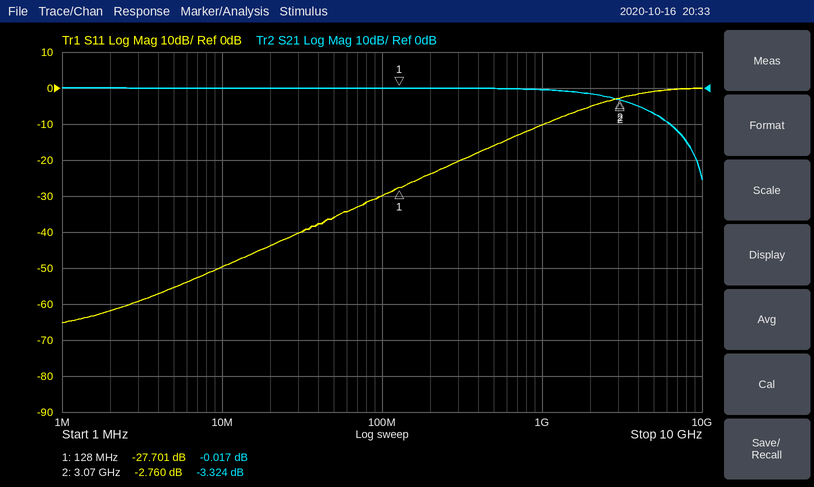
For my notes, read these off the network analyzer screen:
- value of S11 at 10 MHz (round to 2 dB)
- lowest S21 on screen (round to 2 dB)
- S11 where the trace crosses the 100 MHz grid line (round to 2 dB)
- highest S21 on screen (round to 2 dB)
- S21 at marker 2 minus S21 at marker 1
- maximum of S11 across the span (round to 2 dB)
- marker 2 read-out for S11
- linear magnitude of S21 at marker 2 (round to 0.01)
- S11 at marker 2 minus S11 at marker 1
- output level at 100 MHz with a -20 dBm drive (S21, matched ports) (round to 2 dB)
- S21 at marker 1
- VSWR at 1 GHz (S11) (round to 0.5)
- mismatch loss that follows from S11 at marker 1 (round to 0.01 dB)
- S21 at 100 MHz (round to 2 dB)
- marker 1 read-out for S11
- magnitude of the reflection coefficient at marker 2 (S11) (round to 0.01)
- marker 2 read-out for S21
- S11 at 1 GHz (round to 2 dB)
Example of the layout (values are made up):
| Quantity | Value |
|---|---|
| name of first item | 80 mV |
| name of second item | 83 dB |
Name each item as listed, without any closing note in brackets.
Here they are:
| Quantity | Value |
|---|---|
| value of S11 at 10 MHz | -50 dB |
| lowest S21 on screen | -26 dB |
| S11 where the trace crosses the 100 MHz grid line | -30 dB |
| highest S21 on screen | 0 dB |
| S21 at marker 2 minus S21 at marker 1 | -3.307 dB |
| maximum of S11 across the span | 0 dB |
| marker 2 read-out for S11 | -2.760 dB |
| linear magnitude of S21 at marker 2 | 0.68 |
| S11 at marker 2 minus S11 at marker 1 | 24.941 dB |
| output level at 100 MHz with a -20 dBm drive (S21, matched ports) | -20 dBm |
| S21 at marker 1 | -0.017 dB |
| VSWR at 1 GHz (S11) | 2.0 |
| mismatch loss that follows from S11 at marker 1 | 0.01 dB |
| S21 at 100 MHz | 0 dB |
| marker 1 read-out for S11 | -27.701 dB |
| magnitude of the reflection coefficient at marker 2 (S11) | 0.73 |
| marker 2 read-out for S21 | -3.324 dB |
| S11 at 1 GHz | -10 dB |
